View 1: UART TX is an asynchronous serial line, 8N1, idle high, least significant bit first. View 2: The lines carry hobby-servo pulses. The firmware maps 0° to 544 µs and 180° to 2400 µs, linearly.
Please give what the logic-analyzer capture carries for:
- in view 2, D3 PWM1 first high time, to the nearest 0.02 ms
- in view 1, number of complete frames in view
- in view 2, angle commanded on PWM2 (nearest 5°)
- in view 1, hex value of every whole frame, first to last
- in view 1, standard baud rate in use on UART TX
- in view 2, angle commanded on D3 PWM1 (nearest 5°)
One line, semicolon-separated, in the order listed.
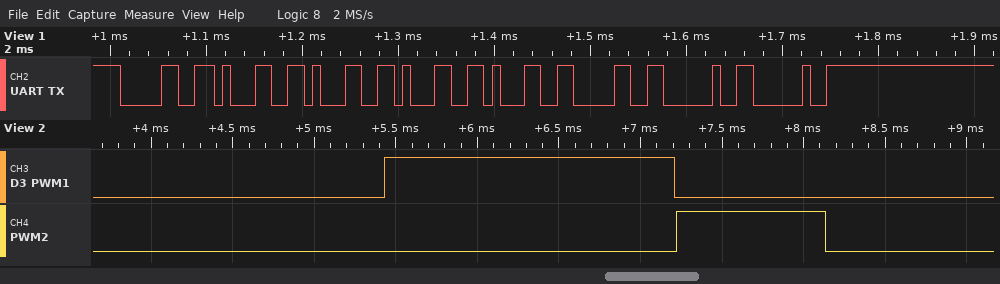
1.78 ms; 8; 35°; 0x30 0x31 0x31 0x31 0x31 0x30 0x20 0x20; 115200 baud; 120°
